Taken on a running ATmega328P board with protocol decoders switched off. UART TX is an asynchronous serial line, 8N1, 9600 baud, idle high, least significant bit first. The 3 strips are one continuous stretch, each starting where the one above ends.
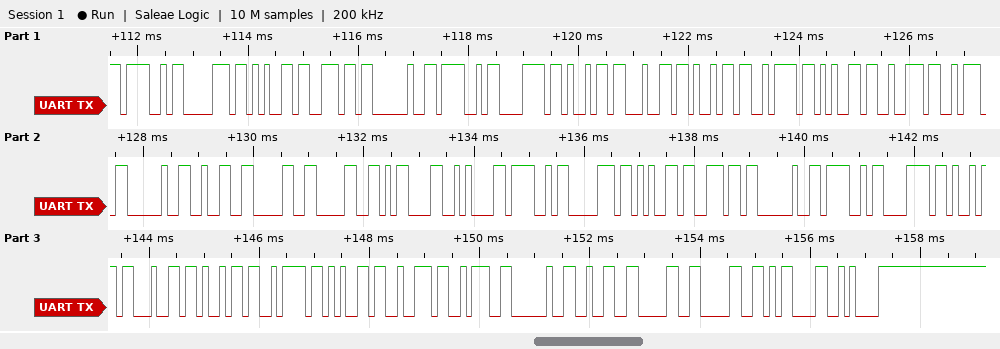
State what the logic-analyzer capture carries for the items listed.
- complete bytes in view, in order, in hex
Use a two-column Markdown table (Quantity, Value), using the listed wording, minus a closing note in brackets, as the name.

| Quantity | Value |
|---|---|
| complete bytes in view, in order, in hex | 4F 70 65 6E 20 4F 78 69 64 69 7A 65 72 3A 20 32 30 30 0D 0A 4F 70 65 6E 20 4F 78 69 64 69 7A 65 72 3A 20 32 30 30 0D 0A |
